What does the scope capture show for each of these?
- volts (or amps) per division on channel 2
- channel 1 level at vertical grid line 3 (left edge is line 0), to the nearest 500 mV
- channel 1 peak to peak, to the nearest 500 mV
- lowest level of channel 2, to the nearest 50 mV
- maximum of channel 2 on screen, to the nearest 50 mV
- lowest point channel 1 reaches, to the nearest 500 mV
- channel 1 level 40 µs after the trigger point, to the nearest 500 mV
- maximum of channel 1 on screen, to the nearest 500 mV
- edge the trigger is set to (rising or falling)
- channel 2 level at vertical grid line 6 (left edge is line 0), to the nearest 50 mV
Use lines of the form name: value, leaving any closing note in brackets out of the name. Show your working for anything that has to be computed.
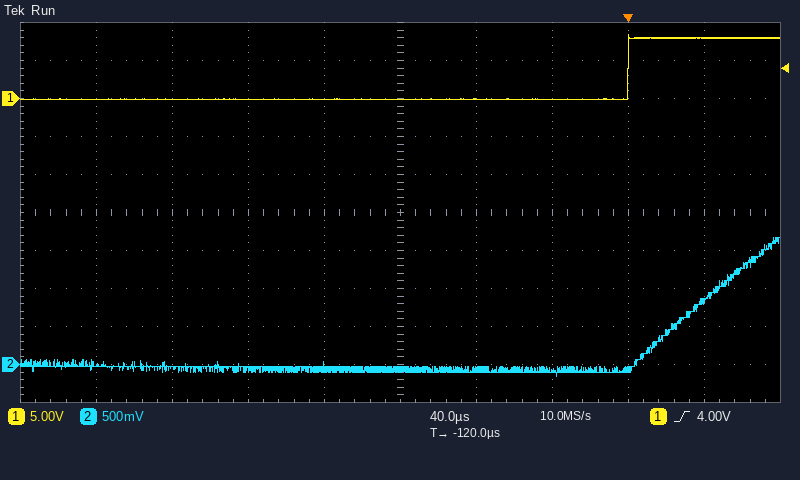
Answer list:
volts (or amps) per division on channel 2: 500 mV
channel 1 level at vertical grid line 3 (left edge is line 0), to the nearest 500 mV: 0.0 V
channel 1 peak to peak, to the nearest 500 mV: 8.5 V − (0.0 V) = 8.5 V
lowest level of channel 2, to the nearest 50 mV: -150 mV
maximum of channel 2 on screen, to the nearest 50 mV: 1.65 V
lowest point channel 1 reaches, to the nearest 500 mV: 0.0 V
channel 1 level 40 µs after the trigger point, to the nearest 500 mV: 8.0 V
maximum of channel 1 on screen, to the nearest 500 mV: 8.5 V
edge the trigger is set to: rising
channel 2 level at vertical grid line 6 (left edge is line 0), to the nearest 50 mV: -50 mV
